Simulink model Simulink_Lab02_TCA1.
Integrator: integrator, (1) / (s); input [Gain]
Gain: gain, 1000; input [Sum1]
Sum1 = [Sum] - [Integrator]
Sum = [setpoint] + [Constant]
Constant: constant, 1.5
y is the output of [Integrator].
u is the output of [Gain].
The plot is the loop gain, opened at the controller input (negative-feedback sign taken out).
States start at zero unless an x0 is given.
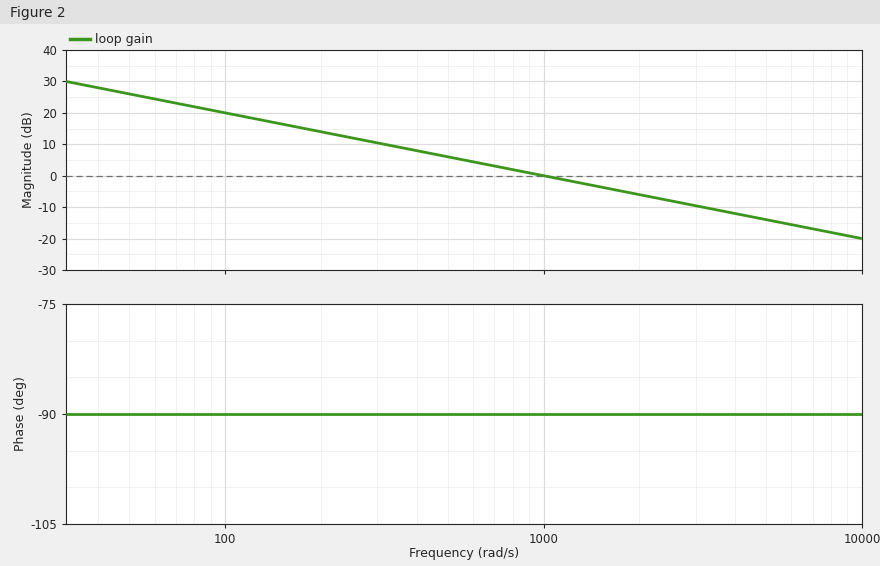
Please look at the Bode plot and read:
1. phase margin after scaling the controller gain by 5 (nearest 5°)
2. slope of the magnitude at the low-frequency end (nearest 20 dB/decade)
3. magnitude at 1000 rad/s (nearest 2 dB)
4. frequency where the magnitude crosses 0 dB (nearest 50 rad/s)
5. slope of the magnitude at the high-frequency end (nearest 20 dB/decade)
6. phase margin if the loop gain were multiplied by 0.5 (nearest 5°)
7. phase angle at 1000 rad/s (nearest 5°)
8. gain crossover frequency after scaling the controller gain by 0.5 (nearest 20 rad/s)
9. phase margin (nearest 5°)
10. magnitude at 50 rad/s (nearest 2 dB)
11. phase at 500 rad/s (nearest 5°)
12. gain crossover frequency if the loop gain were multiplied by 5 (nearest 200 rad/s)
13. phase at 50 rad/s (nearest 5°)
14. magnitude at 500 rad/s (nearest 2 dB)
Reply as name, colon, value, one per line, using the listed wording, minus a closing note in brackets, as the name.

phase margin after scaling the controller gain by 5: 90°
slope of the magnitude at the low-frequency end: -20 dB/decade
magnitude at 1000 rad/s: 0 dB
frequency where the magnitude crosses 0 dB: 1000 rad/s
slope of the magnitude at the high-frequency end: -20 dB/decade
phase margin if the loop gain were multiplied by 0.5: 90°
phase angle at 1000 rad/s: -90°
gain crossover frequency after scaling the controller gain by 0.5: 500 rad/s
phase margin: 90°
magnitude at 50 rad/s: 26 dB
phase at 500 rad/s: -90°
gain crossover frequency if the loop gain were multiplied by 5: 5000 rad/s
phase at 50 rad/s: -90°
magnitude at 500 rad/s: 6 dB
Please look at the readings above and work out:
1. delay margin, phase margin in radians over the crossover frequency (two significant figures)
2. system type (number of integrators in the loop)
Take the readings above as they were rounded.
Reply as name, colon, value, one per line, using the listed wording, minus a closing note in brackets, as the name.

delay margin, phase margin in radians over the crossover frequency: 0.0016 s
system type: 1
